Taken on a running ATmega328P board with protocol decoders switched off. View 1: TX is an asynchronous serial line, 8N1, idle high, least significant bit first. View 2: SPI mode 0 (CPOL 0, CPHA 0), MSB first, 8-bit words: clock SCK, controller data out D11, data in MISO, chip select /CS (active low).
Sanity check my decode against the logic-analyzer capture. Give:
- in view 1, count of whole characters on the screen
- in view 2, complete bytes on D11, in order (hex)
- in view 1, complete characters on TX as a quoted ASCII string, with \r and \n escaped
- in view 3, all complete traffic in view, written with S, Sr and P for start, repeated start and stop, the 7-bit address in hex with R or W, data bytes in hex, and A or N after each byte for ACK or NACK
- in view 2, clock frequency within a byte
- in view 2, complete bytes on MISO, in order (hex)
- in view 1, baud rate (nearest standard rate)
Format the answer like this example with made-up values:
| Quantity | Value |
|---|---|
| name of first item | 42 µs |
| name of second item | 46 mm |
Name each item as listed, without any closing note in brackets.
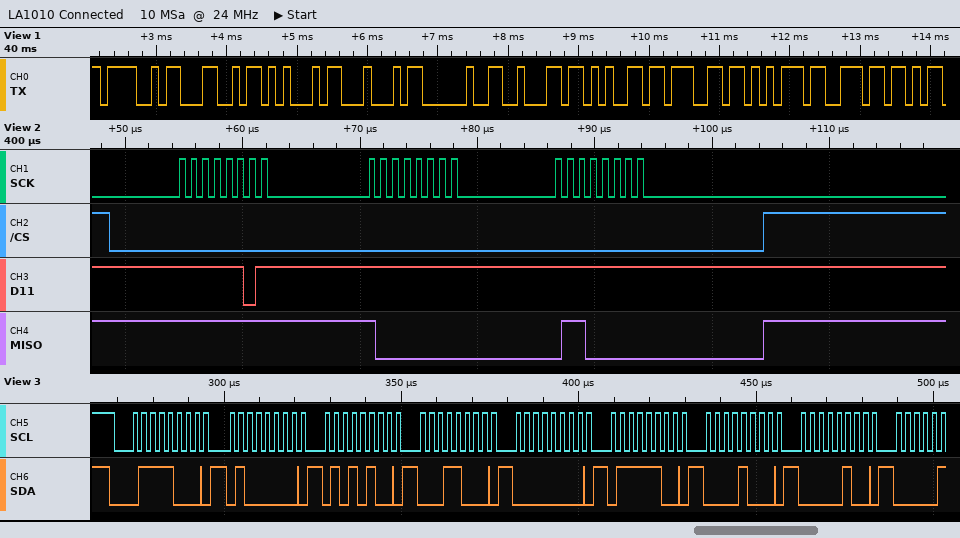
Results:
| Quantity | Value |
|---|---|
| in view 1, count of whole characters on the screen | 10 |
| in view 2, complete bytes on D11, in order | FD FF FF |
| in view 1, complete characters on TX as a quoted ASCII string, with \r and \n escaped | "OLED begun" |
| in view 3, all complete traffic in view, written with S, Sr and P for start, repeated start and stop, the 7-bit address in hex with R or W, data bytes in hex, and A or N after each byte for ACK or NACK | S 3CW A 40 A 54 A 18 A 00 A 7C A 08 A 04 A |
| in view 2, clock frequency within a byte | 1 MHz |
| in view 2, complete bytes on MISO, in order | FF 80 60 |
| in view 1, baud rate | 9600 baud |
